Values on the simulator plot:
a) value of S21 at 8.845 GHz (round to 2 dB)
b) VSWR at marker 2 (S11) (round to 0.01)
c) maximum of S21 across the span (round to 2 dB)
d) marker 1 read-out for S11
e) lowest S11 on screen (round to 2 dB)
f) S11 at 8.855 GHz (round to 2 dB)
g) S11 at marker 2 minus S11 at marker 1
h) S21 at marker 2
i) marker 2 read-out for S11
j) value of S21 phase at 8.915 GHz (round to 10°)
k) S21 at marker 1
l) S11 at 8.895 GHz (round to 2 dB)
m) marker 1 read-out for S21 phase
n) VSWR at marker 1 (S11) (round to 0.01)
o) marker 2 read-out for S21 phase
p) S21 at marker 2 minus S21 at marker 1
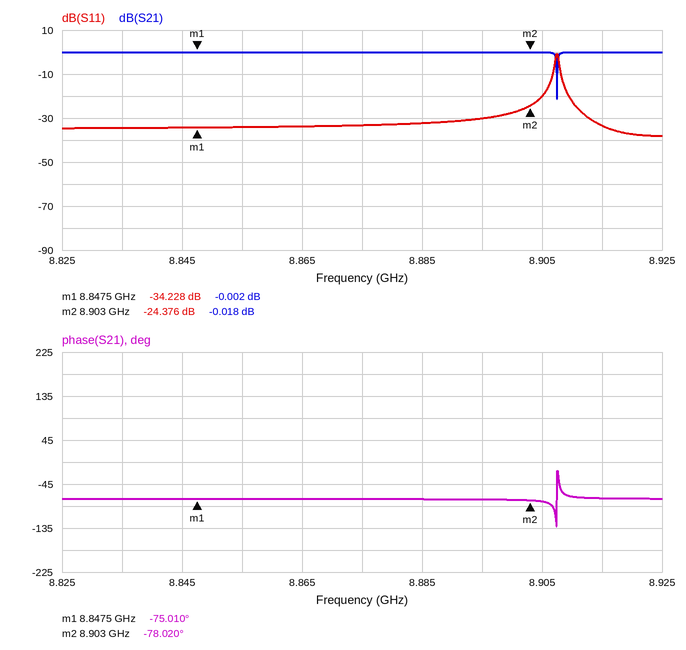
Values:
0 dB
1.13
0 dB
-34.228 dB
-38 dB
-34 dB
9.852 dB
-0.018 dB
-24.376 dB
-70°
-0.002 dB
-30 dB
-75.010°
1.04
-78.020°
-0.016 dB
